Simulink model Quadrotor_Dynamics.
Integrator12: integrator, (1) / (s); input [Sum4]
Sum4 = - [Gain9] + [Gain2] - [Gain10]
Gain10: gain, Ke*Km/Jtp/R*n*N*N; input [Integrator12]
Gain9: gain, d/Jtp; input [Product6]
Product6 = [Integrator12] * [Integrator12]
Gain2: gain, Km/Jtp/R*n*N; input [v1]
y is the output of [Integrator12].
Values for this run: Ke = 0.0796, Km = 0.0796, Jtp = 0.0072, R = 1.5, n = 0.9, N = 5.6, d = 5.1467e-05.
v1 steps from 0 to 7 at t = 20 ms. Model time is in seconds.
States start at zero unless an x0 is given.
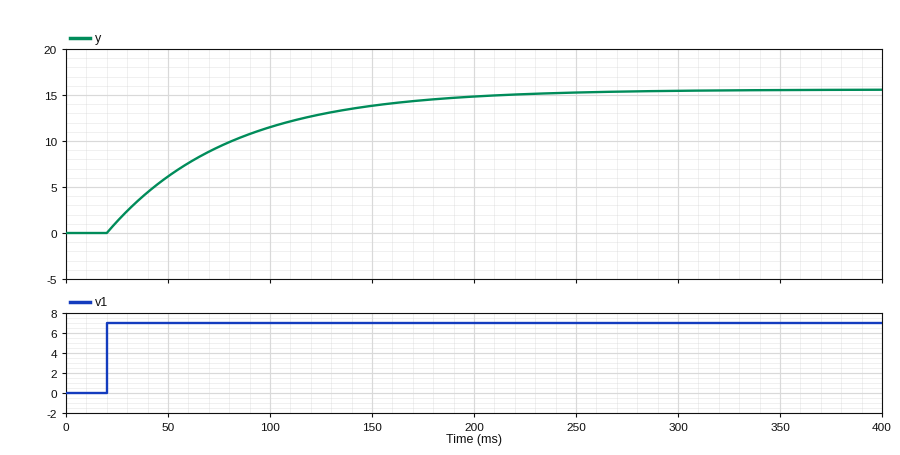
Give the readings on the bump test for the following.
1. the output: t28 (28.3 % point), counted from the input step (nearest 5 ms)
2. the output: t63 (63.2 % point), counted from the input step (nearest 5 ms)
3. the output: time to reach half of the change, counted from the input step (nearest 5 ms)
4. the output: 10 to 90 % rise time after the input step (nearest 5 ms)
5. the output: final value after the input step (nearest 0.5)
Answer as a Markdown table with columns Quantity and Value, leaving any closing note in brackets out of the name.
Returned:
| Quantity | Value |
|---|---|
| the output: t28 (28.3 % point), counted from the input step | 20 ms |
| the output: t63 (63.2 % point), counted from the input step | 60 ms |
| the output: time to reach half of the change, counted from the input step | 40 ms |
| the output: 10 to 90 % rise time after the input step | 130 ms |
| the output: final value after the input step | 15.5 |
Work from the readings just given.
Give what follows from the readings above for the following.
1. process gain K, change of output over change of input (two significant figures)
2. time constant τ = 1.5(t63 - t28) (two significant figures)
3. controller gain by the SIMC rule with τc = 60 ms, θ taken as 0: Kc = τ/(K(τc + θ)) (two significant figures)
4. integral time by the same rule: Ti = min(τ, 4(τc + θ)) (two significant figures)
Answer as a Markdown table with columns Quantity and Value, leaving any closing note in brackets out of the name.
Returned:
| Quantity | Value |
|---|---|
| process gain K, change of output over change of input | 2.2 |
| time constant τ = 1.5(t63 - t28) | 60 ms |
| controller gain by the SIMC rule with τc = 60 ms, θ taken as 0: Kc = τ/(K(τc + θ)) | 0.45 |
| integral time by the same rule: Ti = min(τ, 4(τc + θ)) | 60 ms |
